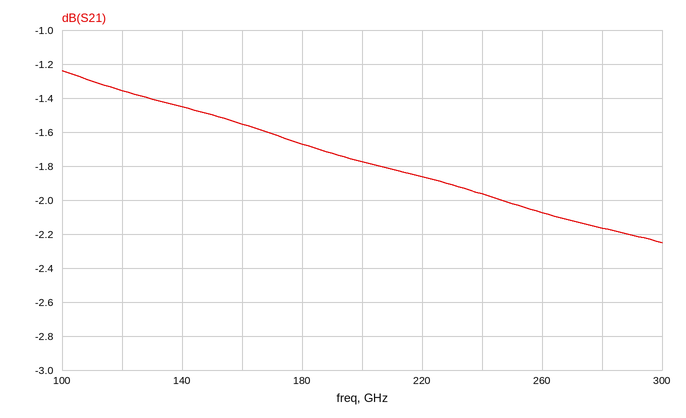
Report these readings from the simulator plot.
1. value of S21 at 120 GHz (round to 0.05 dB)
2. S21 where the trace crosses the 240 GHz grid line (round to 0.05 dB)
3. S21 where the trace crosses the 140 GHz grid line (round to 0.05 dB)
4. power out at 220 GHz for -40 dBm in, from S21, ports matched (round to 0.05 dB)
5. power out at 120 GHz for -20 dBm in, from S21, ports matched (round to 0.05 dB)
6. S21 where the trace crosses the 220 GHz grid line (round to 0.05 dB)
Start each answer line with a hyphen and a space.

- -1.35 dB
- -1.95 dB
- -1.45 dB
- -41.85 dBm
- -21.35 dBm
- -1.85 dB
